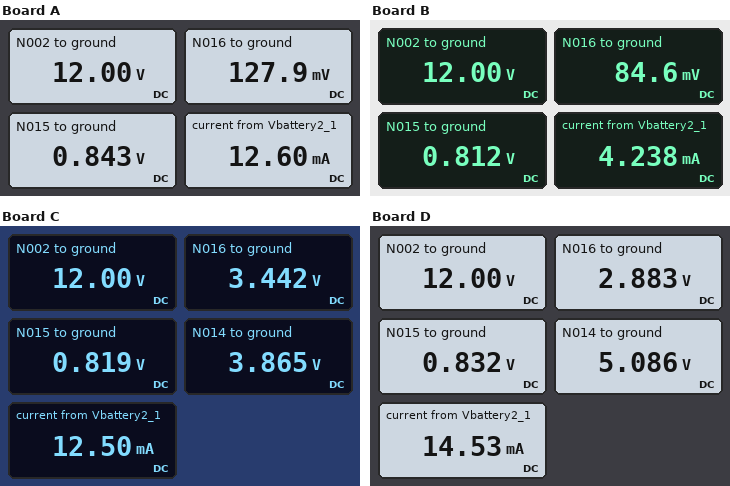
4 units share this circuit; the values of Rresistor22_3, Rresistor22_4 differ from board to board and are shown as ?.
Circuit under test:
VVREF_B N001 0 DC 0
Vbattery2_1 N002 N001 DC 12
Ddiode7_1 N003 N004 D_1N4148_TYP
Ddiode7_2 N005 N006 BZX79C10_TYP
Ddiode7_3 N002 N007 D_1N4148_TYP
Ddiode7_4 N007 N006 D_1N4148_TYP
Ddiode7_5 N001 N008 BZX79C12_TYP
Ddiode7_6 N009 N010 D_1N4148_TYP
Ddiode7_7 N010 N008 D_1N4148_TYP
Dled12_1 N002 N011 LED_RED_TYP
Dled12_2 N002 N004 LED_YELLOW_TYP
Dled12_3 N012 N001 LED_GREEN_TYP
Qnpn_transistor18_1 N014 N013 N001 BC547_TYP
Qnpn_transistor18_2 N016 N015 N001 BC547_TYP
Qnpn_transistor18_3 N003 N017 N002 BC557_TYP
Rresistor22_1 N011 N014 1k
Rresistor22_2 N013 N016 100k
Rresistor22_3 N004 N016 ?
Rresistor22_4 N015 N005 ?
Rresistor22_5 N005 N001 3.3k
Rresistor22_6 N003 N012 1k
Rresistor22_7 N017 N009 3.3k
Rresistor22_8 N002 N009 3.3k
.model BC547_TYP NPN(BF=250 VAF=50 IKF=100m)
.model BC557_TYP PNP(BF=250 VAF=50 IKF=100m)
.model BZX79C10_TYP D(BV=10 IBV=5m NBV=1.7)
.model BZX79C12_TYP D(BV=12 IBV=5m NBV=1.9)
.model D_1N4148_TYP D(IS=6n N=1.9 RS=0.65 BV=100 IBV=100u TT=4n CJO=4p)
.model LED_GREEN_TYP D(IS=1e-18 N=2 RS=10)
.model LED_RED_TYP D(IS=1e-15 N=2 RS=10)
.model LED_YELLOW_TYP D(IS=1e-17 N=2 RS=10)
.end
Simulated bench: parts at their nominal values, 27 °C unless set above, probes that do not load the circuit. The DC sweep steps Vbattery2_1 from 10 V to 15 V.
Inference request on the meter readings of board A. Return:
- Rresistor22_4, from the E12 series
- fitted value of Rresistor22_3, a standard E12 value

1 kΩ
820 Ω
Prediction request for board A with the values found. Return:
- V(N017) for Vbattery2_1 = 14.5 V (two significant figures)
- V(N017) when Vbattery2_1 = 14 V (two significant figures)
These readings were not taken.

14 V
13 V
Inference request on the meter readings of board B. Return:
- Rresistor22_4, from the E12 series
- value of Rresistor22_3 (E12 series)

1 kΩ
2.7 kΩ
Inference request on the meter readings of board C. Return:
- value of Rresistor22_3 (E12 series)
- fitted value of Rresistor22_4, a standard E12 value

1.2 kΩ
10 kΩ
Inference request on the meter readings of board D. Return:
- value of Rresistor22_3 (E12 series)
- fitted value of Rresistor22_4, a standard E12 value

820 Ω
5.6 kΩ
